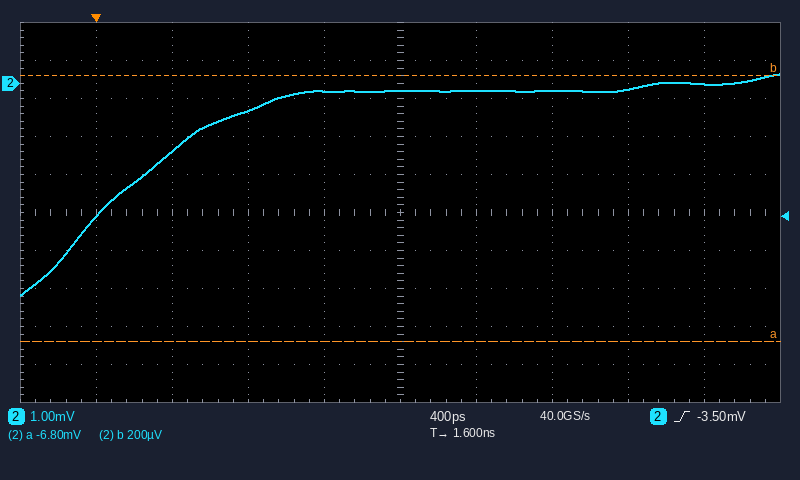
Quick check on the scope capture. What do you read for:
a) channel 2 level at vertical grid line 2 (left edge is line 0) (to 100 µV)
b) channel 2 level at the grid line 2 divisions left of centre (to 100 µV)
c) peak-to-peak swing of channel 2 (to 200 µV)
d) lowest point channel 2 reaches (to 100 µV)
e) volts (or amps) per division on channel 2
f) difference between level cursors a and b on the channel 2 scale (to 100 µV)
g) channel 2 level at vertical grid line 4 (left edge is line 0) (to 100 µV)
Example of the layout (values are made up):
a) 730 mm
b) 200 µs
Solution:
a) -1.8 mV
b) -700 µV
c) 5.8 mV
d) -5.6 mV
e) 1 mV
f) 7.0 mV
g) -200 µV
